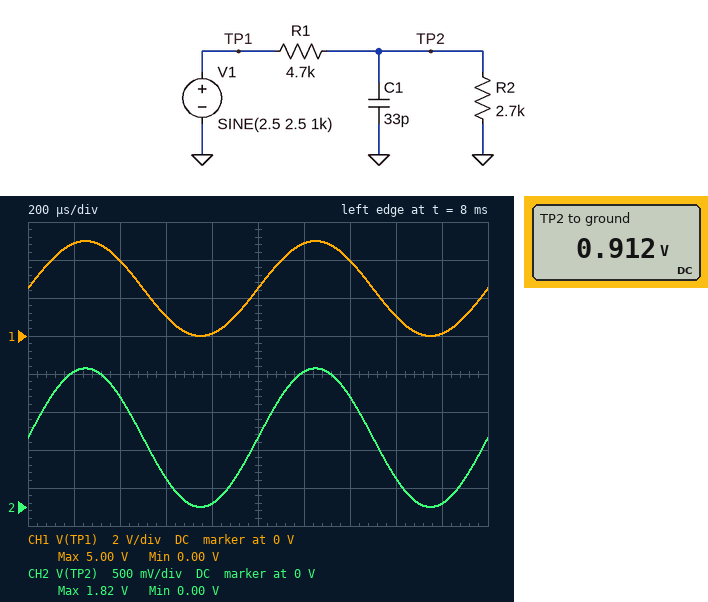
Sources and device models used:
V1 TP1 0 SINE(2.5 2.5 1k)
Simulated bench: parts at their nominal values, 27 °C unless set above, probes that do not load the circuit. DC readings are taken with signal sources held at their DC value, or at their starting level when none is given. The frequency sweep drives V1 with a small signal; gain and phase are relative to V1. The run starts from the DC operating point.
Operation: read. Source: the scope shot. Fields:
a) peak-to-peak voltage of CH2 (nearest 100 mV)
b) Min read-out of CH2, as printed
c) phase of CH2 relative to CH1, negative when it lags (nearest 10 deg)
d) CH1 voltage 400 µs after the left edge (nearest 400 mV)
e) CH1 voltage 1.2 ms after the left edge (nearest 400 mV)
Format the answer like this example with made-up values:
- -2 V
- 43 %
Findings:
- 1.8 V
- 0.00 V
- 0 deg
- 4.0 V
- 4.8 V
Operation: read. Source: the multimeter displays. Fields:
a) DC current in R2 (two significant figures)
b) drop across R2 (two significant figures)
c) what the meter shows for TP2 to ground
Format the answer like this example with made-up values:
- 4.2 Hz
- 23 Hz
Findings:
- 340 µA
- 910 mV
- 0.912 V
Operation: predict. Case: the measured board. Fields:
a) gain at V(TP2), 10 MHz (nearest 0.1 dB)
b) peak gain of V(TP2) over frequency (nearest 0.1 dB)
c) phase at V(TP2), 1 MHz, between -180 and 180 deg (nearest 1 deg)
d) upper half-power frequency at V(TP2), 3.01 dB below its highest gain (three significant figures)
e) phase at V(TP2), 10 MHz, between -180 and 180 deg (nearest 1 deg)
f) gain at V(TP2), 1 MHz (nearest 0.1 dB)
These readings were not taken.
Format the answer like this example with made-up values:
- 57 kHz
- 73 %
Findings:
- -20.1 dB
- -8.8 dB
- -20 deg
- 2.81 MHz
- -74 deg
- -9.3 dB
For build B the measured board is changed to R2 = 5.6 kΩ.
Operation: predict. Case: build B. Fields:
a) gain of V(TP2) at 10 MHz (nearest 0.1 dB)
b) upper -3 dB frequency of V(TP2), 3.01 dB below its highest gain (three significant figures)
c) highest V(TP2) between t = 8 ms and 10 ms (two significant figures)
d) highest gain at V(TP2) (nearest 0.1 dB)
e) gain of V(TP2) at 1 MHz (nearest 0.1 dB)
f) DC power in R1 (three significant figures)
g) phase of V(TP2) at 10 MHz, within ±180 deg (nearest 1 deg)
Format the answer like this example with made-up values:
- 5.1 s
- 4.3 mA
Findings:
- -19.9 dB
- 1.89 MHz
- 2.7 V
- -5.3 dB
- -6.4 dB
- 277 µW
- -79 deg
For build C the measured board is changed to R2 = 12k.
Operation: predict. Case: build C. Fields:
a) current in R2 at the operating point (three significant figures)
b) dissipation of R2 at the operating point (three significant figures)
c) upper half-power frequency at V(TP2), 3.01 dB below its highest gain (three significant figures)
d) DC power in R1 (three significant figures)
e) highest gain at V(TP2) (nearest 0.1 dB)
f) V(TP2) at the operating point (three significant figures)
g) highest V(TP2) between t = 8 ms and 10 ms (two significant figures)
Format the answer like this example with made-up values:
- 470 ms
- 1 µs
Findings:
- 150 µA
- 269 µW
- 1.43 MHz
- 105 µW
- -2.9 dB
- 1.80 V
- 3.6 V
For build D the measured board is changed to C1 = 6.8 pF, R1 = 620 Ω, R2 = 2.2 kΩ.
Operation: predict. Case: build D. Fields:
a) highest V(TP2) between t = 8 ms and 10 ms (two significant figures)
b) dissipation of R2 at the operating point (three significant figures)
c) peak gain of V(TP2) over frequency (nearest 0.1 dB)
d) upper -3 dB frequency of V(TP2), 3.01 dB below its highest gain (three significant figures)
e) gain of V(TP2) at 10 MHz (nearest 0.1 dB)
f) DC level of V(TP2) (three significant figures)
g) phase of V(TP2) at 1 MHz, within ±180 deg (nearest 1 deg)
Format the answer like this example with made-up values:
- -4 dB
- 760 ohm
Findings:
- 3.9 V
- 1.73 mW
- -2.2 dB
- 48.4 MHz
- -2.3 dB
- 1.95 V
- -1 deg
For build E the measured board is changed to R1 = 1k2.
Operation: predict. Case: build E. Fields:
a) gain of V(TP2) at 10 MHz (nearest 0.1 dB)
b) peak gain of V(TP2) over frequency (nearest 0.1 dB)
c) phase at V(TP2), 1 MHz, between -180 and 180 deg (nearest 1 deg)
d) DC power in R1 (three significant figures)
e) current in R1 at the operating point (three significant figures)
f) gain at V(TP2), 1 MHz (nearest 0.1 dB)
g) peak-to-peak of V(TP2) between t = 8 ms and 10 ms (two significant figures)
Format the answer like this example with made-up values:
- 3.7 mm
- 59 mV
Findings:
- -9.2 dB
- -3.2 dB
- -10 deg
- 493 µW
- 641 µA
- -3.3 dB
- 3.5 V
